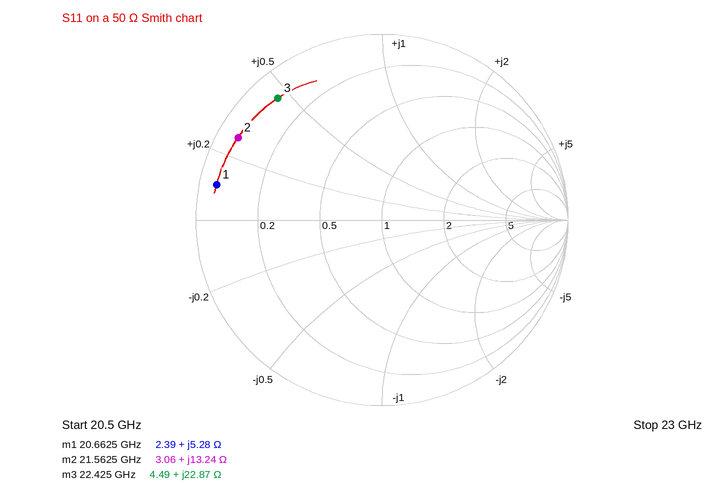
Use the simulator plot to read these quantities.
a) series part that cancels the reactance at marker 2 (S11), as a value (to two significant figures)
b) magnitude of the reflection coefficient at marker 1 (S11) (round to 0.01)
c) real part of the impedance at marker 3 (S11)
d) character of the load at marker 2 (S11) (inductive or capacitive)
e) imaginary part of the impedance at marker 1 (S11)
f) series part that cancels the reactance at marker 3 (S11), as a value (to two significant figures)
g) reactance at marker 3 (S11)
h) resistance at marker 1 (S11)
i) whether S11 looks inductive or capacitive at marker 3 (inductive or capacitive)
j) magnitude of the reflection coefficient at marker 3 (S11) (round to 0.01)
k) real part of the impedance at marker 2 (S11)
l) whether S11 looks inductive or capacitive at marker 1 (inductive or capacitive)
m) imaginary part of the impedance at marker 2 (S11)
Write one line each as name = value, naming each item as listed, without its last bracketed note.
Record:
series part that cancels the reactance at marker 2 (S11), as a value = 560 fF
magnitude of the reflection coefficient at marker 1 (S11) = 0.91
real part of the impedance at marker 3 = 4.49 Ω
character of the load at marker 2 (S11) = inductive
imaginary part of the impedance at marker 1 = +5.28 Ω
series part that cancels the reactance at marker 3 (S11), as a value = 310 fF
reactance at marker 3 = +22.87 Ω
resistance at marker 1 = 2.39 Ω
whether S11 looks inductive or capacitive at marker 3 = inductive
magnitude of the reflection coefficient at marker 3 (S11) = 0.86
real part of the impedance at marker 2 = 3.06 Ω
whether S11 looks inductive or capacitive at marker 1 = inductive
imaginary part of the impedance at marker 2 = +13.24 Ω
